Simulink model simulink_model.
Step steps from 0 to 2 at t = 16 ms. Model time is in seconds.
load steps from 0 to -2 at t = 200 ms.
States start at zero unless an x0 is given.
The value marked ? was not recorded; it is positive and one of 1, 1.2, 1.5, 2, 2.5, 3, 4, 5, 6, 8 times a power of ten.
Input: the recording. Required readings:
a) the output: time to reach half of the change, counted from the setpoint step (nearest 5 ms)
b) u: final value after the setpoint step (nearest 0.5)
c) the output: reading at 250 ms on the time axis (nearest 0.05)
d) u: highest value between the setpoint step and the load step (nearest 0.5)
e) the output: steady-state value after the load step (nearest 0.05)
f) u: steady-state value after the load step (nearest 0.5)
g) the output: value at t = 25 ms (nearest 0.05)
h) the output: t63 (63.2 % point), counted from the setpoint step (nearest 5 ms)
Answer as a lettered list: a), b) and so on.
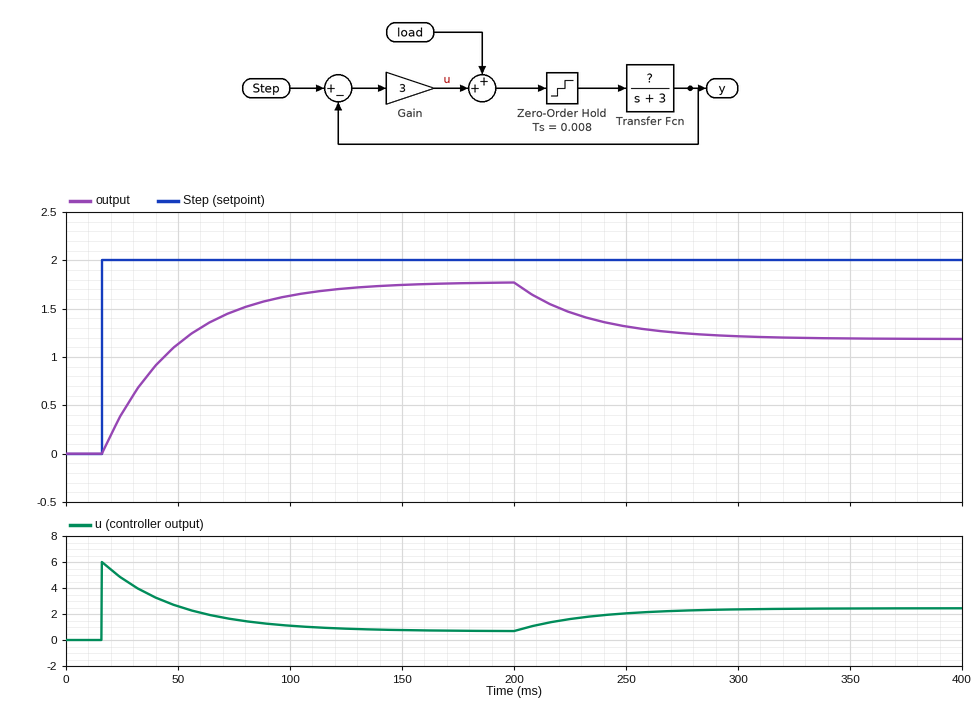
a) 25 ms
b) 0.5
c) 1.30
d) 6.0
e) 1.20
f) 2.5
g) 0.40
h) 35 ms
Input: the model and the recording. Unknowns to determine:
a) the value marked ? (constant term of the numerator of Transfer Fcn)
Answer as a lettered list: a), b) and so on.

a) 8
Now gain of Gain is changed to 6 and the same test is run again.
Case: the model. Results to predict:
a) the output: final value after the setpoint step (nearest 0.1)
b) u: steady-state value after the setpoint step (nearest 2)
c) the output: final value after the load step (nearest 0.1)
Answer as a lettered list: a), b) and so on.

a) 1.9
b) 0
c) 1.6
